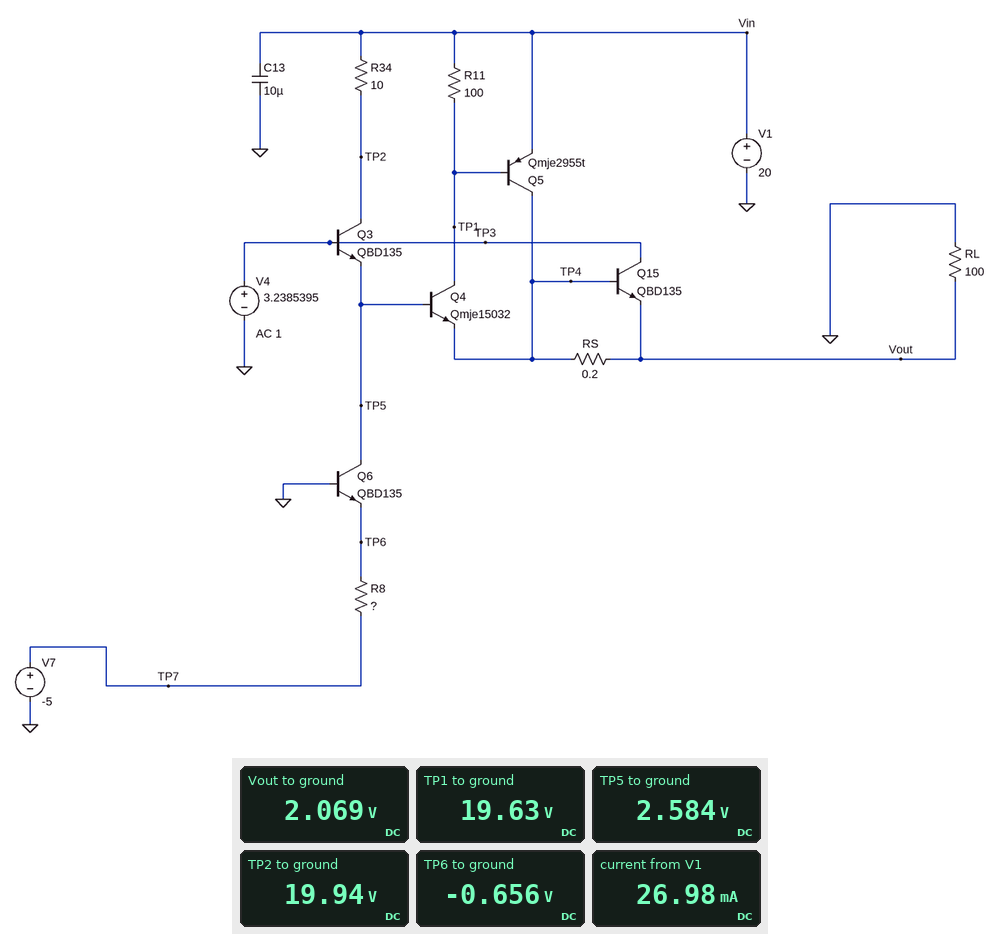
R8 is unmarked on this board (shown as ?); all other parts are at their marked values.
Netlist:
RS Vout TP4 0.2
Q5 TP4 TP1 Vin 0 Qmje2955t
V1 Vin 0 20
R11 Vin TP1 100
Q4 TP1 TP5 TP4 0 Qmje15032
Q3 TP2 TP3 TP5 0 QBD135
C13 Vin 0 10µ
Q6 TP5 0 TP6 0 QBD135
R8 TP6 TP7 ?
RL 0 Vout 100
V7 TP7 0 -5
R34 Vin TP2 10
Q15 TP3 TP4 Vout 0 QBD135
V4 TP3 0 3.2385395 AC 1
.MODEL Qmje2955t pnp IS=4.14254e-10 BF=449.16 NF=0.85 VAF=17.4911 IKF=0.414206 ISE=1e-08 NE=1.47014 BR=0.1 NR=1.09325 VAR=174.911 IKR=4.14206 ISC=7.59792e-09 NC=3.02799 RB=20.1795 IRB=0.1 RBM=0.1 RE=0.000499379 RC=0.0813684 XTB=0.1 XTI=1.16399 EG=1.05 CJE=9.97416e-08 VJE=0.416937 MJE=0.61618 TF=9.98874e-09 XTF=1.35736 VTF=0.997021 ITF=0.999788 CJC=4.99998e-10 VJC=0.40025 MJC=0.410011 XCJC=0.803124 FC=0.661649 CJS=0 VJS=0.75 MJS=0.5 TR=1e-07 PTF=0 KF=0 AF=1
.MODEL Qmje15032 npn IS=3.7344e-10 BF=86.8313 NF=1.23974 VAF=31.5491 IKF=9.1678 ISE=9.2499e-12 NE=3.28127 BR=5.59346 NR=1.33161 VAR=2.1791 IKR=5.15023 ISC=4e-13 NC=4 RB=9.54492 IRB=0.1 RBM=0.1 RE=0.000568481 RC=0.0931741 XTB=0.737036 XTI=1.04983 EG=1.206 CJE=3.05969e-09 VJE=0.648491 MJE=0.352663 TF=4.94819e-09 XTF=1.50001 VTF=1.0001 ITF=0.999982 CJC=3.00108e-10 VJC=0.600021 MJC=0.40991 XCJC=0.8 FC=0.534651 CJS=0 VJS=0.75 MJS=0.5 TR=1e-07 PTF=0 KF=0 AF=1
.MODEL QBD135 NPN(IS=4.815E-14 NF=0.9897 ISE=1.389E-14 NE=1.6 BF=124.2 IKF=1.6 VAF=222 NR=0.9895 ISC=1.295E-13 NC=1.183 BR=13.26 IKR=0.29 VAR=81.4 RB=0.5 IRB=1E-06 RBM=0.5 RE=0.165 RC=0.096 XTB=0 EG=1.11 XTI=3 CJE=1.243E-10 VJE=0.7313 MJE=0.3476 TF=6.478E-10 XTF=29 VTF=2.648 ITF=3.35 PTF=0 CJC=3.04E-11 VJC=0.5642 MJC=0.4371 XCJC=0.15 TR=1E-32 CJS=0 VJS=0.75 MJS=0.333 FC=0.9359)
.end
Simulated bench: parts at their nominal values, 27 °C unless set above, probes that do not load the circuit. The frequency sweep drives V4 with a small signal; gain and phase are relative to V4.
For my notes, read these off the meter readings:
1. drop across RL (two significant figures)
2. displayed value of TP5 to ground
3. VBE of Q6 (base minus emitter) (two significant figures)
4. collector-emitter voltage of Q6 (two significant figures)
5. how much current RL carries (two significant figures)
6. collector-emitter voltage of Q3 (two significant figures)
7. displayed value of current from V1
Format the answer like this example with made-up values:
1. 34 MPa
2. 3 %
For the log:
1. 2.1 V
2. 2.584 V
3. 660 mV
4. 3.2 V
5. 21 mA
6. 17 V
7. 26.98 mA
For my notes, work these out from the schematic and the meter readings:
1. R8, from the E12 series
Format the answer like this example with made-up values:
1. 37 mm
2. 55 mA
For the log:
1. 680 Ω
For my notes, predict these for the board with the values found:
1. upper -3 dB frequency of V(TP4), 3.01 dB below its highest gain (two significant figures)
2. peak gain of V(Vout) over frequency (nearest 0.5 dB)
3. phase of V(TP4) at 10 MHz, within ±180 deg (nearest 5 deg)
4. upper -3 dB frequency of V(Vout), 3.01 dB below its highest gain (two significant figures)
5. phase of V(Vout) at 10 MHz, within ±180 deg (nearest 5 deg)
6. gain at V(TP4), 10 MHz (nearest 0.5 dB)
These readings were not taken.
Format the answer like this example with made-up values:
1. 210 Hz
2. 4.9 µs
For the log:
1. 39 MHz
2. 0 dB
3. -10 deg
4. 39 MHz
5. -10 deg
6. -1.5 dB
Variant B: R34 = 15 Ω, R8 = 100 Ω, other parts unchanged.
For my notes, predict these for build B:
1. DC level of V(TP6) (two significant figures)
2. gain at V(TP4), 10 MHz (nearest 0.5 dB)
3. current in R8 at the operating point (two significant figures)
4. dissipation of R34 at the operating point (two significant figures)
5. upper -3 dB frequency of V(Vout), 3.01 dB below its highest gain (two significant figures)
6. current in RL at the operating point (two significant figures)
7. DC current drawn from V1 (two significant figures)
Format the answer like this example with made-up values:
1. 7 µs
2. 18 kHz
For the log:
1. -710 mV
2. -1.0 dB
3. 43 mA
4. 27 mW
5. 59 MHz
6. 20 mA
7. 62 mA
